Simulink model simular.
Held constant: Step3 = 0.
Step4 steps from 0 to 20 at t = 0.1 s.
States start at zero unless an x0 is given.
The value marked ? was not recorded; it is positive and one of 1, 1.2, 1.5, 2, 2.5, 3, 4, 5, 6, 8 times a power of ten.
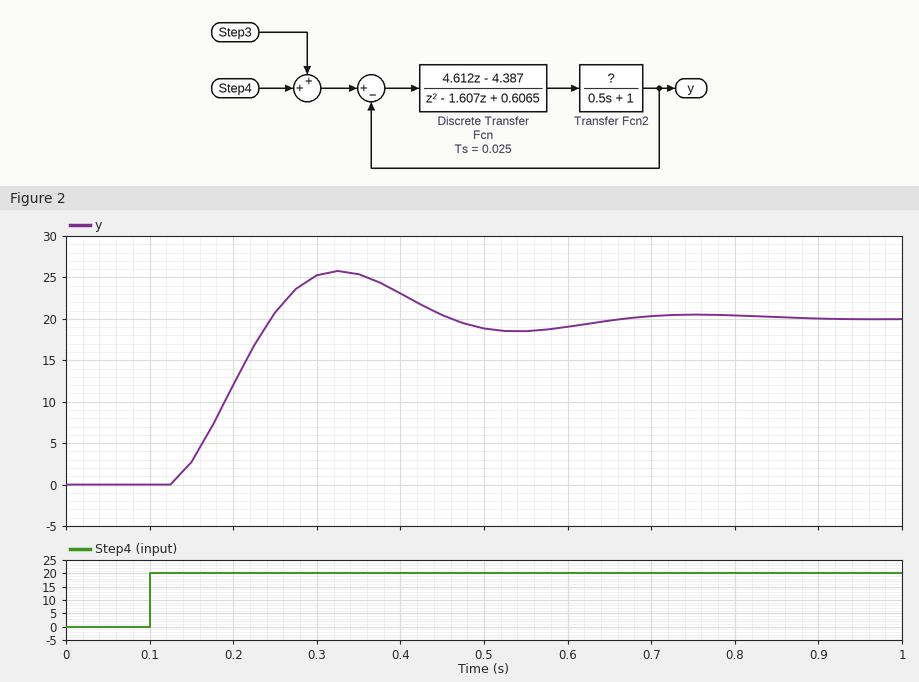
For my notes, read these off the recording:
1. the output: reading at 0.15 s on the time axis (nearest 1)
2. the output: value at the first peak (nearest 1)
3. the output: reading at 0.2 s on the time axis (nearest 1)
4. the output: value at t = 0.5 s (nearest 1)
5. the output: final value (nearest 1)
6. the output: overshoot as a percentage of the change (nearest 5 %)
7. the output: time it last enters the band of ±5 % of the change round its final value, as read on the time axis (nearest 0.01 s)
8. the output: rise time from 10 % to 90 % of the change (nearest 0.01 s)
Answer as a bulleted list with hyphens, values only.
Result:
- 3
- 26
- 12
- 19
- 20
- 30 %
- 0.60 s
- 0.09 s
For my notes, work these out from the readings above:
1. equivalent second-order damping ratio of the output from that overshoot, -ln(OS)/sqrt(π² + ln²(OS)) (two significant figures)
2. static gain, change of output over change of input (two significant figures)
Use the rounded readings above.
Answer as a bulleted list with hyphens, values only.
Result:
- 0.36
- 1.0
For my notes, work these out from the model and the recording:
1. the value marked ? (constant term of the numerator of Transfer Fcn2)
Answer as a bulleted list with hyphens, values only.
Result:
- 0.6
